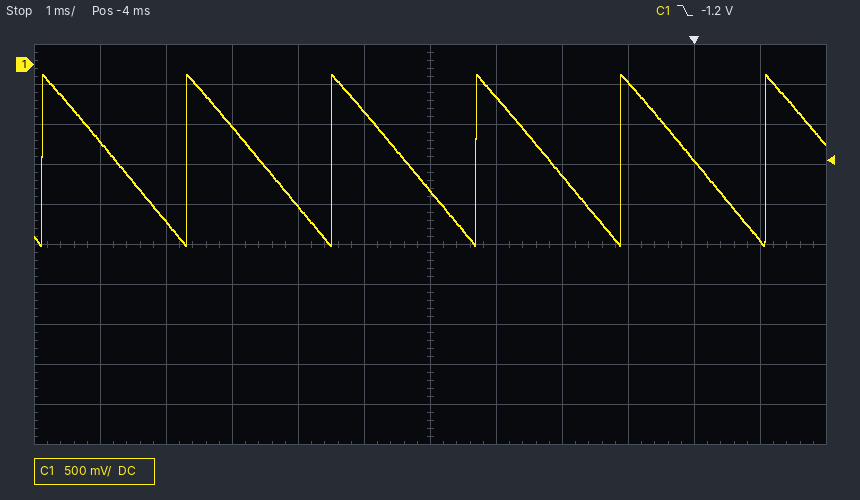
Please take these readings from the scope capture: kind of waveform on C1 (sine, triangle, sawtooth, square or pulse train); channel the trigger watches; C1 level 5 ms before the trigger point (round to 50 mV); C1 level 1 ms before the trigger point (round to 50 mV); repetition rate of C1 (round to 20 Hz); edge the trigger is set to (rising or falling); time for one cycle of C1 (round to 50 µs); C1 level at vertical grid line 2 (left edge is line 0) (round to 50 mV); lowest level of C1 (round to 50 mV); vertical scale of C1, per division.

sawtooth
C1
-600 mV
-200 mV
460 Hz
falling
2.20 ms
-1.95 V
-2.25 V
500 mV
